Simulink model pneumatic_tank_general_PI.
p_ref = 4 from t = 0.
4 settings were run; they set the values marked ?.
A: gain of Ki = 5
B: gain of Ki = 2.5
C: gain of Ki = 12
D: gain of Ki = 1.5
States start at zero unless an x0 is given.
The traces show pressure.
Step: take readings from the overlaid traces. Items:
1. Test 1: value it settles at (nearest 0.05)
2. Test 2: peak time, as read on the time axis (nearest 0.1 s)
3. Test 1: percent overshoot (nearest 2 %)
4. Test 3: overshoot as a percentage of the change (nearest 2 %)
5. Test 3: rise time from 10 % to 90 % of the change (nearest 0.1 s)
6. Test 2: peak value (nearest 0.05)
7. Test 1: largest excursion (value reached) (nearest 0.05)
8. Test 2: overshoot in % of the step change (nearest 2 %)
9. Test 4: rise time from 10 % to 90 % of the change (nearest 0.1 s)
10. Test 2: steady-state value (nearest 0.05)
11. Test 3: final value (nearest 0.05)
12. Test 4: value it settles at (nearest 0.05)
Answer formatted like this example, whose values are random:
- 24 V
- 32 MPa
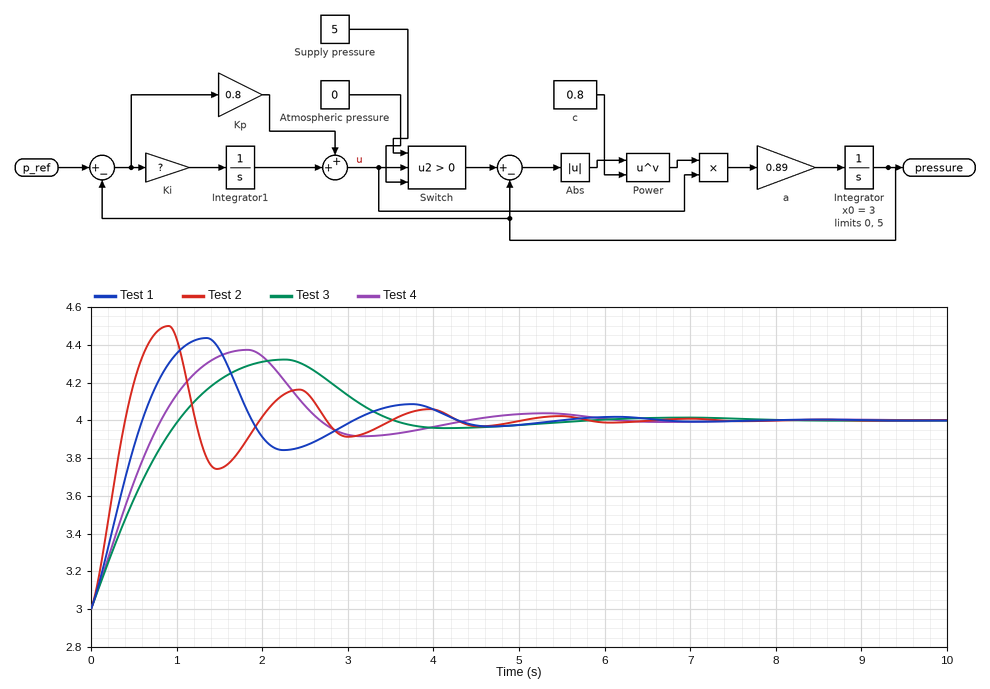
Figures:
- 4.00
- 0.9 s
- 44 %
- 32 %
- 0.8 s
- 4.50
- 4.45
- 50 %
- 0.6 s
- 4.00
- 4.00
- 4.00
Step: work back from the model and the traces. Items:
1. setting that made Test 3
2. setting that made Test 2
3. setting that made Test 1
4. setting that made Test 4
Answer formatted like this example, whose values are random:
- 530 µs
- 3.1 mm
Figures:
- D
- C
- A
- B
